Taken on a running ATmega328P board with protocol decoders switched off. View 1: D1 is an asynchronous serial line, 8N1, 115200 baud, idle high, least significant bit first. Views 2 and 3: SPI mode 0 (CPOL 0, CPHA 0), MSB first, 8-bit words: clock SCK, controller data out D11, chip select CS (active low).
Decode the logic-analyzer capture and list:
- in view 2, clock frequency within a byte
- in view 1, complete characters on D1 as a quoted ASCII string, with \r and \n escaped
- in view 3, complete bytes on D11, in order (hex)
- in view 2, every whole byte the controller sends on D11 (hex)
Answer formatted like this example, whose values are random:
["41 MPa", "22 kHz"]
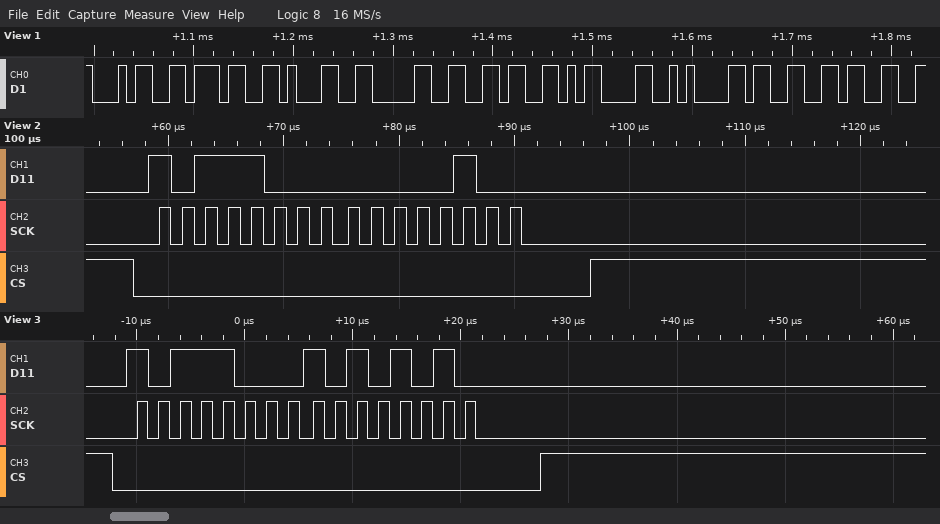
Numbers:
["500 kHz", "\"47106\\r\\n33\"", "B8 AA", "0xB8 0x04"]
